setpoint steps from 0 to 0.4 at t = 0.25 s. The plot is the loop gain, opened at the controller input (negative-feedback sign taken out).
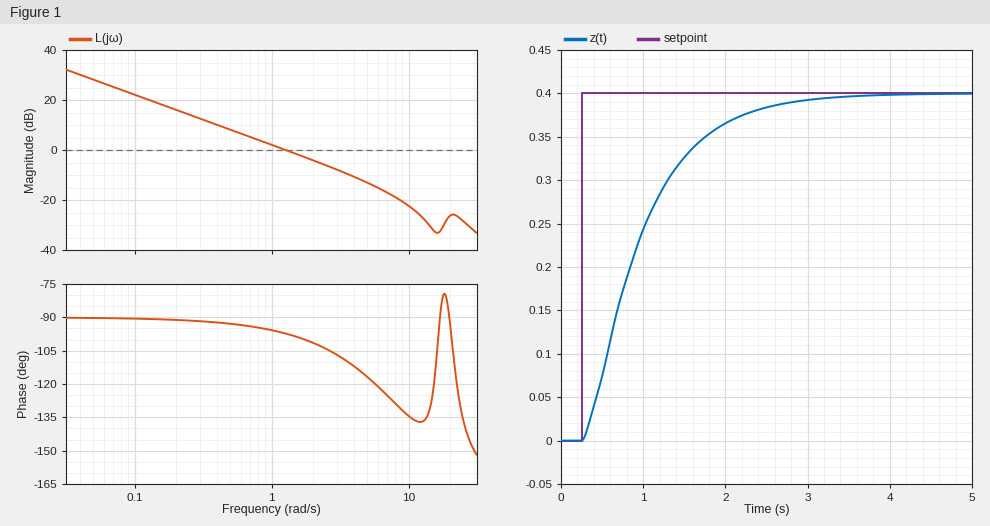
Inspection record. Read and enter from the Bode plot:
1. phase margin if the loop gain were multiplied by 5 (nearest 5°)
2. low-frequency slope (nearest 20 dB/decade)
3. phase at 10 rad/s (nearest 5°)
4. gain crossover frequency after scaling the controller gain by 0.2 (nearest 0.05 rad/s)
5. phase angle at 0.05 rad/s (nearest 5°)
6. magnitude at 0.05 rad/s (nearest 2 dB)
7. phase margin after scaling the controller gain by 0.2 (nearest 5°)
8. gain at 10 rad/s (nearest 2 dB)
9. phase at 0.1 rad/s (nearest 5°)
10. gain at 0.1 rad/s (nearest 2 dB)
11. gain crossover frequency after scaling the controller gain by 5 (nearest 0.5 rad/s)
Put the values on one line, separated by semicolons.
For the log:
60°; -20 dB/decade; -135°; 0.25 rad/s; -90°; 28 dB; 90°; -22 dB; -90°; 22 dB; 5.5 rad/s
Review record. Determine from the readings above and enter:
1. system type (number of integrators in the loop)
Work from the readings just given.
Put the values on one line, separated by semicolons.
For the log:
1
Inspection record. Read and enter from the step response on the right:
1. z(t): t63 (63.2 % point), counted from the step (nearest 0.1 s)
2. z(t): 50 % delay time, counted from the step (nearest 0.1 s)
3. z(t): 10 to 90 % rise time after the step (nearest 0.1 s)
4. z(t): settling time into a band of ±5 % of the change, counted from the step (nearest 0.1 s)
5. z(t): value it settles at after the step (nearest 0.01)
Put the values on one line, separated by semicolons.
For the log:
0.8 s; 0.6 s; 1.5 s; 2.1 s; 0.40
